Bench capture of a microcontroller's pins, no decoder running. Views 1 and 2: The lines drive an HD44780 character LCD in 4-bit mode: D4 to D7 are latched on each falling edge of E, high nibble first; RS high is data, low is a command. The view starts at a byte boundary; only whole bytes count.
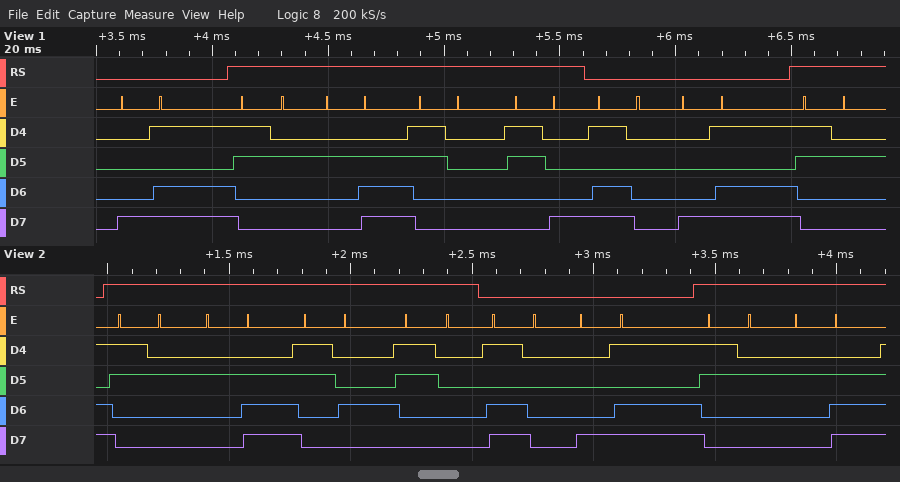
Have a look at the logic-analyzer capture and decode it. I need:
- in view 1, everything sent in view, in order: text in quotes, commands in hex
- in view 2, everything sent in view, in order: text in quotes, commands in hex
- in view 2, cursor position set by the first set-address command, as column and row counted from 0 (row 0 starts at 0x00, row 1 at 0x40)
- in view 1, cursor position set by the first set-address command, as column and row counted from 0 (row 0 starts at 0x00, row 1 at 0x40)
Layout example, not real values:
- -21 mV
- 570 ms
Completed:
- 0x8D "2.08" 0xD0 0x8D "2"
- "2.40" 0xD0 0x8D "2."
- column 16, row 1
- column 13, row 0
